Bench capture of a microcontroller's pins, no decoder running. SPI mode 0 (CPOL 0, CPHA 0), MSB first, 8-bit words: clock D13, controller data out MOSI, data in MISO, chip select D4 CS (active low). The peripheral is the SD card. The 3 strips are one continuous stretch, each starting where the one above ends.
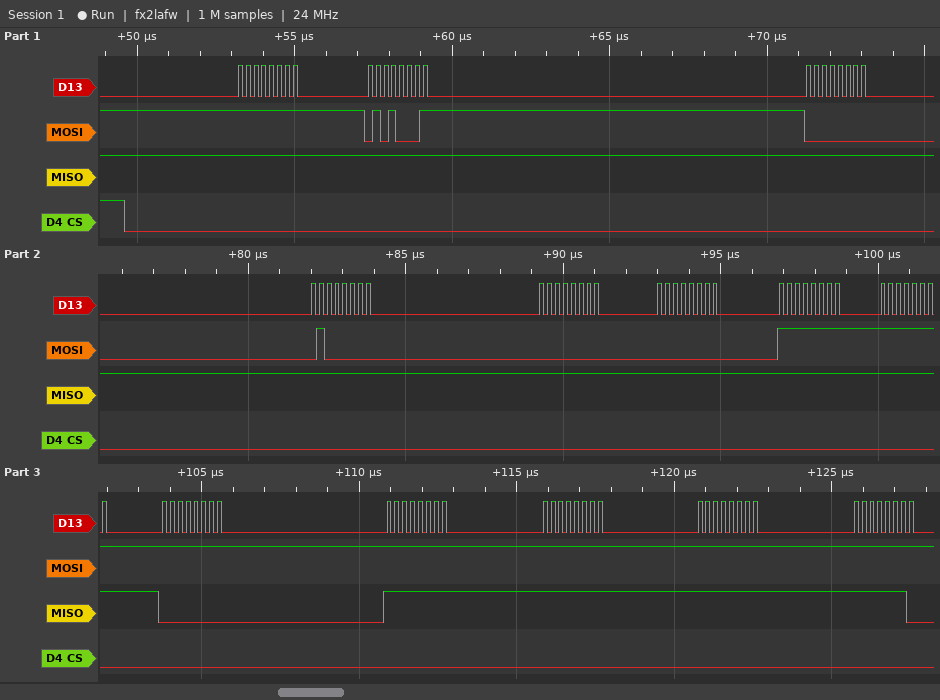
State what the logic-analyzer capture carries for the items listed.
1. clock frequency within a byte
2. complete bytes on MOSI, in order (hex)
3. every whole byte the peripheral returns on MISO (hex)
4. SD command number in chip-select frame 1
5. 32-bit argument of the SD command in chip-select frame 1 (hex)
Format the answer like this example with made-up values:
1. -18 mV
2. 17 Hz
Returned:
1. 4 MHz
2. 0xFF 0x51 0x00 0x40 0x00 0x00 0xFF 0xFF 0xFF 0xFF 0xFF 0xFF 0xFF
3. 0xFF 0xFF 0xFF 0xFF 0xFF 0xFF 0xFF 0xFF 0x00 0xFF 0xFF 0xFF 0xFE
4. CMD17
5. 0x00400000
